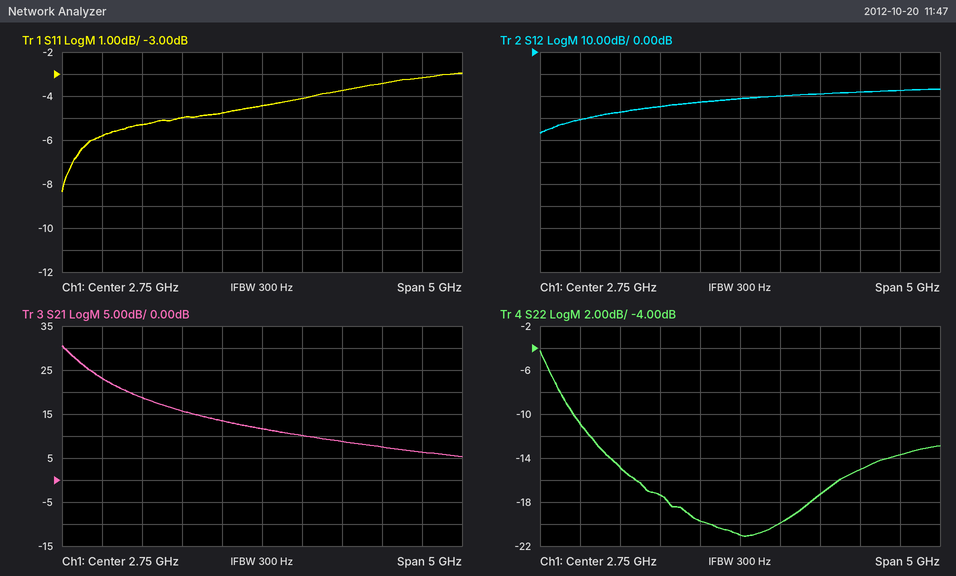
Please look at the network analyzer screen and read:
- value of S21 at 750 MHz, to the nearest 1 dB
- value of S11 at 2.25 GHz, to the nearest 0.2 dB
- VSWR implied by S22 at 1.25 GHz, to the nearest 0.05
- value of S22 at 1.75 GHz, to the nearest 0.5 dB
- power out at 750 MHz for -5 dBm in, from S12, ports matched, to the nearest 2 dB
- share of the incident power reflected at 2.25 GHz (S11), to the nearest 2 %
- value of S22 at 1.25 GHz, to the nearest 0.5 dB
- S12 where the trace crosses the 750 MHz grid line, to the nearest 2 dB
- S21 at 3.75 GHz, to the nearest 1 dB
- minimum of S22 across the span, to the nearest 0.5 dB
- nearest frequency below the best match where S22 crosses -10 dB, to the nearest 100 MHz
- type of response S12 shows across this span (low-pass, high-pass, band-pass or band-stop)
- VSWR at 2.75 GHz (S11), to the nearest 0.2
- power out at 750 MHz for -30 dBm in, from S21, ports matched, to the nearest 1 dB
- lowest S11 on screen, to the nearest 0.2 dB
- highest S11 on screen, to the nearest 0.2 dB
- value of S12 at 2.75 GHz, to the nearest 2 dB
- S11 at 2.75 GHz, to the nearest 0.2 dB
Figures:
23 dB
-4.8 dB
1.45
-17.5 dB
-36 dBm
34 %
-15.0 dB
-30 dB
9 dB
-21.0 dB
700 MHz
high-pass
4.0
-7 dBm
-8.4 dB
-3.0 dB
-22 dB
-4.4 dB
